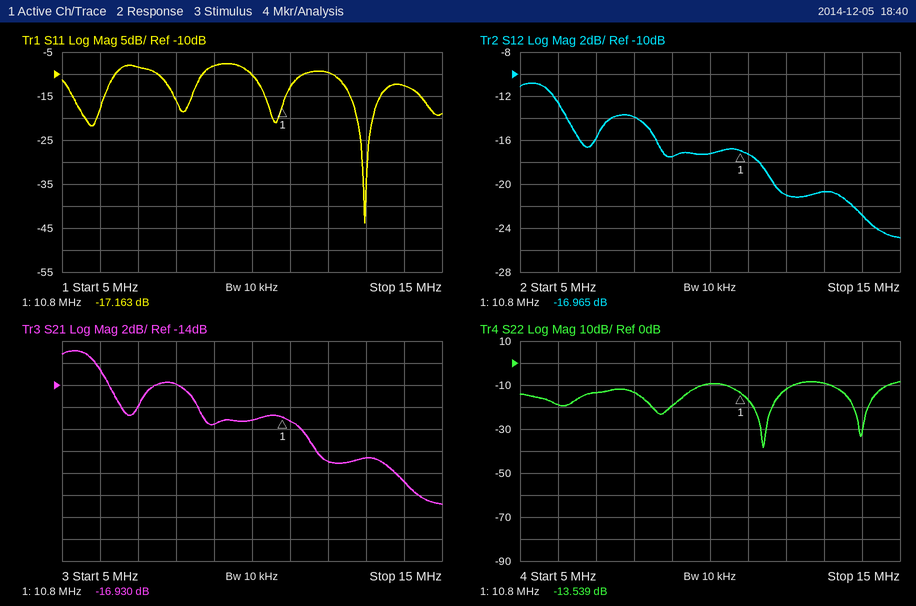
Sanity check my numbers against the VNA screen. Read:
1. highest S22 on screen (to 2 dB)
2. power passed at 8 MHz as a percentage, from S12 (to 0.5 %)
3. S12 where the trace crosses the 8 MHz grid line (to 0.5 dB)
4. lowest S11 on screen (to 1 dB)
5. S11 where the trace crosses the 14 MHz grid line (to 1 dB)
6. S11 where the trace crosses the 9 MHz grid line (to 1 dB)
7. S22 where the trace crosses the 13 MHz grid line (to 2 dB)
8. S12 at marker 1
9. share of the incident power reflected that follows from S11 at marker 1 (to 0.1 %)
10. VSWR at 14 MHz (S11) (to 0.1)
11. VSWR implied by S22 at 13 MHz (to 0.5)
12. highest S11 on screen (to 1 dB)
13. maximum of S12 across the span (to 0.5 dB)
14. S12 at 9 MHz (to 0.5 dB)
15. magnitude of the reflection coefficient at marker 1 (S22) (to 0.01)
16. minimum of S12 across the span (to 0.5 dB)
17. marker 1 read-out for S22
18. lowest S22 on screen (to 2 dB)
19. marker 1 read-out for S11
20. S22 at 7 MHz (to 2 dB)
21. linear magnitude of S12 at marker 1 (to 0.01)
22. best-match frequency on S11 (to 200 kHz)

-8 dB
4.0 %
-14.0 dB
-44 dB
-13 dB
-8 dB
-10 dB
-16.965 dB
1.9 %
1.6
2.0
-8 dB
-11.0 dB
-17.5 dB
0.21
-25.0 dB
-13.539 dB
-38 dB
-17.163 dB
-14 dB
0.14
13.0 MHz
